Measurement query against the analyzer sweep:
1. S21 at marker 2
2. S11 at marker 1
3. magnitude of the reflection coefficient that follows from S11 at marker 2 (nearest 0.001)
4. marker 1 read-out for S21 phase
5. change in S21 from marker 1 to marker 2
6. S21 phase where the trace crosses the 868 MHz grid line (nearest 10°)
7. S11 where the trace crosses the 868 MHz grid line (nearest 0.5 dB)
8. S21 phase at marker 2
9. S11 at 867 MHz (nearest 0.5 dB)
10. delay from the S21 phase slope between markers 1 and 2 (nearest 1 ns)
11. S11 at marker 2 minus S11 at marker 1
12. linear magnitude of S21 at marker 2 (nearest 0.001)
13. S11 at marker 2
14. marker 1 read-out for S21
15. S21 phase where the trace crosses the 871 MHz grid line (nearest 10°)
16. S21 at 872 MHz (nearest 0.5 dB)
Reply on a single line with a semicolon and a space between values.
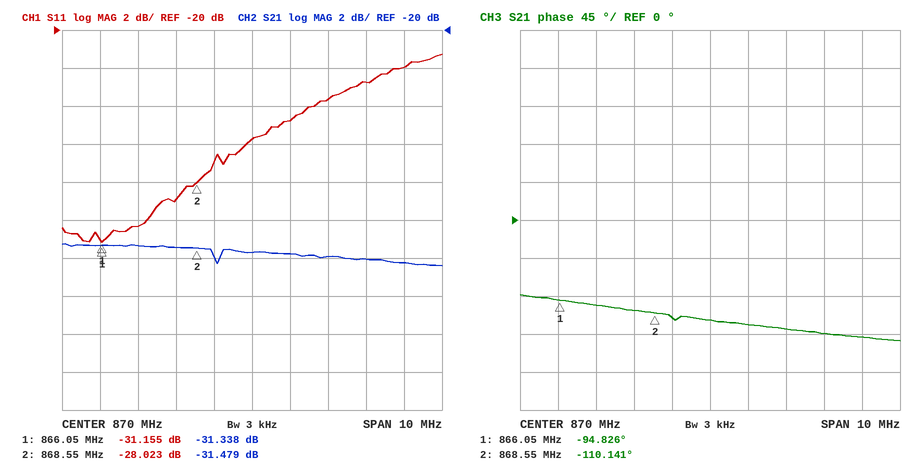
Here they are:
-31.479 dB; -31.155 dB; 0.040; -94.826°; -0.141 dB; -110°; -29.0 dB; -110.141°; -30.5 dB; 17 ns; 3.132 dB; 0.027; -28.023 dB; -31.338 dB; -120°; -32.0 dB
